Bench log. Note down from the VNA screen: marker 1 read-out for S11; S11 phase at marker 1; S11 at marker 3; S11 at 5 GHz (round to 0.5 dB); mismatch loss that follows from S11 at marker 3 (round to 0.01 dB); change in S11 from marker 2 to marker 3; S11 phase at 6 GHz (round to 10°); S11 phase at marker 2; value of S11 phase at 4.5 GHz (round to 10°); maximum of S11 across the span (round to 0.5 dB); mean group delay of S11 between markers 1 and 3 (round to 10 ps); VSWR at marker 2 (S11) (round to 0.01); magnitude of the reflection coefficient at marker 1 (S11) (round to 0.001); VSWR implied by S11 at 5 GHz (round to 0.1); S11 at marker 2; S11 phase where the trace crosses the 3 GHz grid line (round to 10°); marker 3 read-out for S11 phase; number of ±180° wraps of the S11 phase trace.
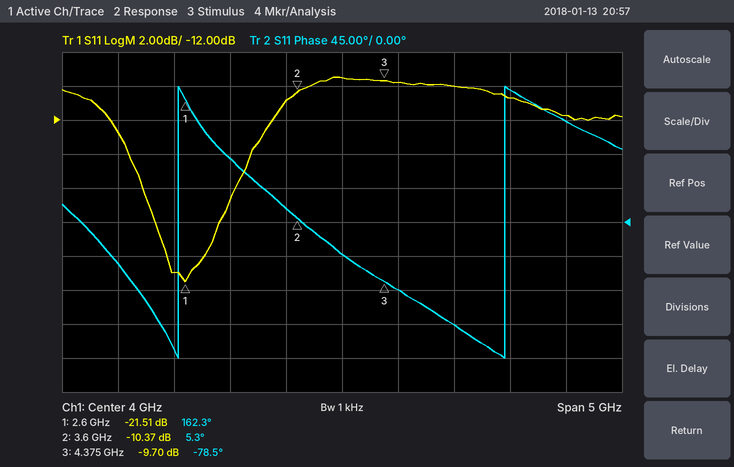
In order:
-21.51 dB
162.3°
-9.70 dB
-10.0 dB
0.49 dB
0.67 dB
130°
5.3°
-90°
-9.5 dB
380 ps
1.87
0.084
1.9
-10.37 dB
80°
-78.5°
2
